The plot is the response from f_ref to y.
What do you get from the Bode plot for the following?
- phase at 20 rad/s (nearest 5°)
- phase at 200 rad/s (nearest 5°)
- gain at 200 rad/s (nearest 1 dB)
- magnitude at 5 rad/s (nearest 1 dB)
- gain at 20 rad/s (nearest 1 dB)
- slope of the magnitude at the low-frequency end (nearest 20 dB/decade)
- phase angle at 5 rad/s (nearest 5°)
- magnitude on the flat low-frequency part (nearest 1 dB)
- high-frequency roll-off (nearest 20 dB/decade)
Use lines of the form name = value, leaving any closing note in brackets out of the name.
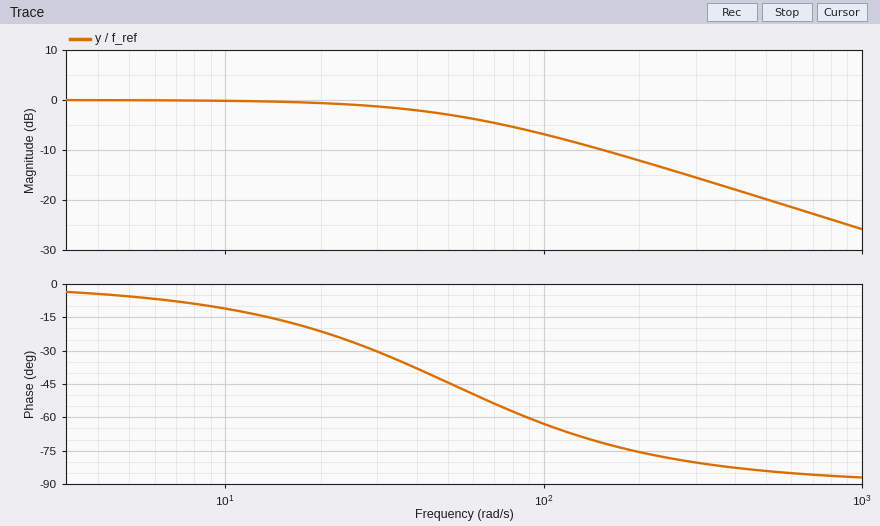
phase at 20 rad/s = -20°
phase at 200 rad/s = -75°
gain at 200 rad/s = -12 dB
magnitude at 5 rad/s = 0 dB
gain at 20 rad/s = -1 dB
slope of the magnitude at the low-frequency end = 0 dB/decade
phase angle at 5 rad/s = -5°
magnitude on the flat low-frequency part = 0 dB
high-frequency roll-off = -20 dB/decade
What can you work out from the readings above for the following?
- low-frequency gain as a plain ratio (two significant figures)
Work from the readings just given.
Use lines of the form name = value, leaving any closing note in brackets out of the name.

low-frequency gain as a plain ratio = 1.0
